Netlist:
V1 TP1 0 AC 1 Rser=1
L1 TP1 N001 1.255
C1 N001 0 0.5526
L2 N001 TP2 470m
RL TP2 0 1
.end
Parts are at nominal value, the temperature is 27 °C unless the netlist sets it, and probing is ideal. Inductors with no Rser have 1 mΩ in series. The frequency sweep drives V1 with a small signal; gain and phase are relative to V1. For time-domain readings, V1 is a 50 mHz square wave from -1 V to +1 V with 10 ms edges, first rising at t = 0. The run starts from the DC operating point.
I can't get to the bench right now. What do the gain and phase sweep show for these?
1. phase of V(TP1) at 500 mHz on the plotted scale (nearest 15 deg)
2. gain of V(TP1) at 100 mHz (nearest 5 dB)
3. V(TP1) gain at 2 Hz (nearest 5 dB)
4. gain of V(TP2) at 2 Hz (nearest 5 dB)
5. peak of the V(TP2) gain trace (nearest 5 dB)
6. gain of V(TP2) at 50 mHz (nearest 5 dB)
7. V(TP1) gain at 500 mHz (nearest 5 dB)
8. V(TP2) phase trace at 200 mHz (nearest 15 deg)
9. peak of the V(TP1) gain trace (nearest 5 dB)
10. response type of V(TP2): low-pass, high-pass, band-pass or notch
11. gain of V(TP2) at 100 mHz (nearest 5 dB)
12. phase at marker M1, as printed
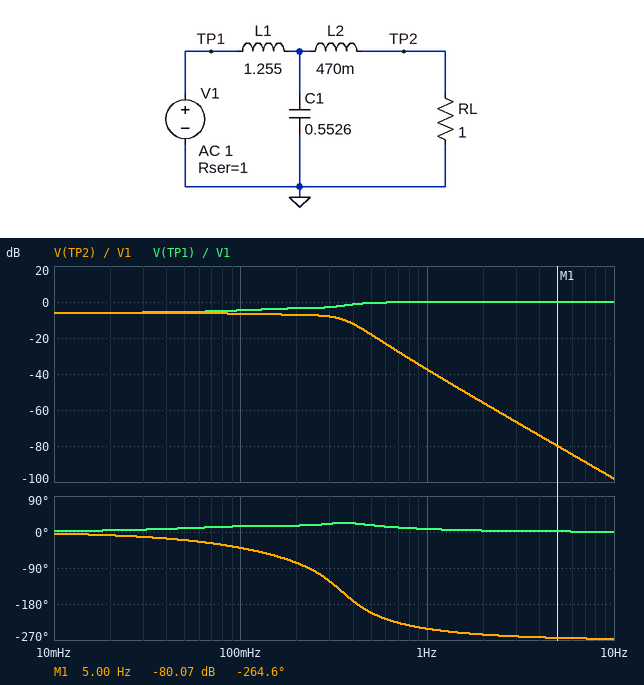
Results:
15 deg
-5 dB
0 dB
-55 dB
-5 dB
-5 dB
0 dB
-75 deg
0 dB
low-pass
-5 dB
-264.6 deg
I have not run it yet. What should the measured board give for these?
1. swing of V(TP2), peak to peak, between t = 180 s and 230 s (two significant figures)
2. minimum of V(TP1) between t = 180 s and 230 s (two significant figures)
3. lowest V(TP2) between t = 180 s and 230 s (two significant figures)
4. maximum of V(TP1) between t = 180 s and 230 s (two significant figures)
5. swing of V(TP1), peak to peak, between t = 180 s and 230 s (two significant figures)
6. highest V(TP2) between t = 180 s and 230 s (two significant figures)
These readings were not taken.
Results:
1.1 V
-1.5 V
-530 mV
1.5 V
3.0 V
530 mV
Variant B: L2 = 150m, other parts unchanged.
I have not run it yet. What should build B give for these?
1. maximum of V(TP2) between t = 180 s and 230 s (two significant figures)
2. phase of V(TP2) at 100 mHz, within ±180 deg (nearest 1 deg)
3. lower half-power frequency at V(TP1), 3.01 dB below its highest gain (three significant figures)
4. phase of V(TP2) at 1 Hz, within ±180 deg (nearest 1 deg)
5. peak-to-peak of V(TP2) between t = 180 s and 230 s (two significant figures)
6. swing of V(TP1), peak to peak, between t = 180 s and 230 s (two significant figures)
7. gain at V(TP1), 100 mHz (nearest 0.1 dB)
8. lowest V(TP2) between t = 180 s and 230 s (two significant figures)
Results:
510 mV
-35 deg
237 mHz
155 deg
1.0 V
3.0 V
-5.3 dB
-510 mV
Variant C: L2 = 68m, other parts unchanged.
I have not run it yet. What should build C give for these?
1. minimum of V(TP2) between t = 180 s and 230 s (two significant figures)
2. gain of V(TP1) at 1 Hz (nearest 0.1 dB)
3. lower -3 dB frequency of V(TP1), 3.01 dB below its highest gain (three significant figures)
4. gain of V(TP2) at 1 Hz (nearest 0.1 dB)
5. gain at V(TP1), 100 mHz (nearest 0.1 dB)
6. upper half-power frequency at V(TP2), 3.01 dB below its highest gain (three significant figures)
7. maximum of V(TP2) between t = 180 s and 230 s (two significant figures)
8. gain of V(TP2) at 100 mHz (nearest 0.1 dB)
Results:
-520 mV
-0.1 dB
235 mHz
-28.6 dB
-5.5 dB
257 mHz
520 mV
-6.3 dB
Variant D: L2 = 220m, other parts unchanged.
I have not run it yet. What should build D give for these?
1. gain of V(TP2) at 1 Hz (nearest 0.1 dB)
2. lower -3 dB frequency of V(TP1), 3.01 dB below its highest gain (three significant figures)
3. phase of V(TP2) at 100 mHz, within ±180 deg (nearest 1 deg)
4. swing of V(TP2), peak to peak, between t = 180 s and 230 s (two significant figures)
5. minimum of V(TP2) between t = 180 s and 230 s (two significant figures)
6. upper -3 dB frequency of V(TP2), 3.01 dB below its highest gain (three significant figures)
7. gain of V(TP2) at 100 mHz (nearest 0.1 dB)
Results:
-31.9 dB
240 mHz
-36 deg
1.0 V
-510 mV
286 mHz
-6.4 dB
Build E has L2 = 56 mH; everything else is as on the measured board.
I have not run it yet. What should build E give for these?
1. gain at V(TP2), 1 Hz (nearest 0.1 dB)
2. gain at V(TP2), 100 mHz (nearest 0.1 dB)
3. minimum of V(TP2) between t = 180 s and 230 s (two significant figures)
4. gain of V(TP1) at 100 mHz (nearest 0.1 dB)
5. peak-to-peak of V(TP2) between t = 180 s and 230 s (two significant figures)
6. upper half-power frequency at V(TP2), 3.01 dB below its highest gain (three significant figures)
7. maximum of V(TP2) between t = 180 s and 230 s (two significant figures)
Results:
-28.5 dB
-6.3 dB
-520 mV
-5.6 dB
1.0 V
255 mHz
520 mV
